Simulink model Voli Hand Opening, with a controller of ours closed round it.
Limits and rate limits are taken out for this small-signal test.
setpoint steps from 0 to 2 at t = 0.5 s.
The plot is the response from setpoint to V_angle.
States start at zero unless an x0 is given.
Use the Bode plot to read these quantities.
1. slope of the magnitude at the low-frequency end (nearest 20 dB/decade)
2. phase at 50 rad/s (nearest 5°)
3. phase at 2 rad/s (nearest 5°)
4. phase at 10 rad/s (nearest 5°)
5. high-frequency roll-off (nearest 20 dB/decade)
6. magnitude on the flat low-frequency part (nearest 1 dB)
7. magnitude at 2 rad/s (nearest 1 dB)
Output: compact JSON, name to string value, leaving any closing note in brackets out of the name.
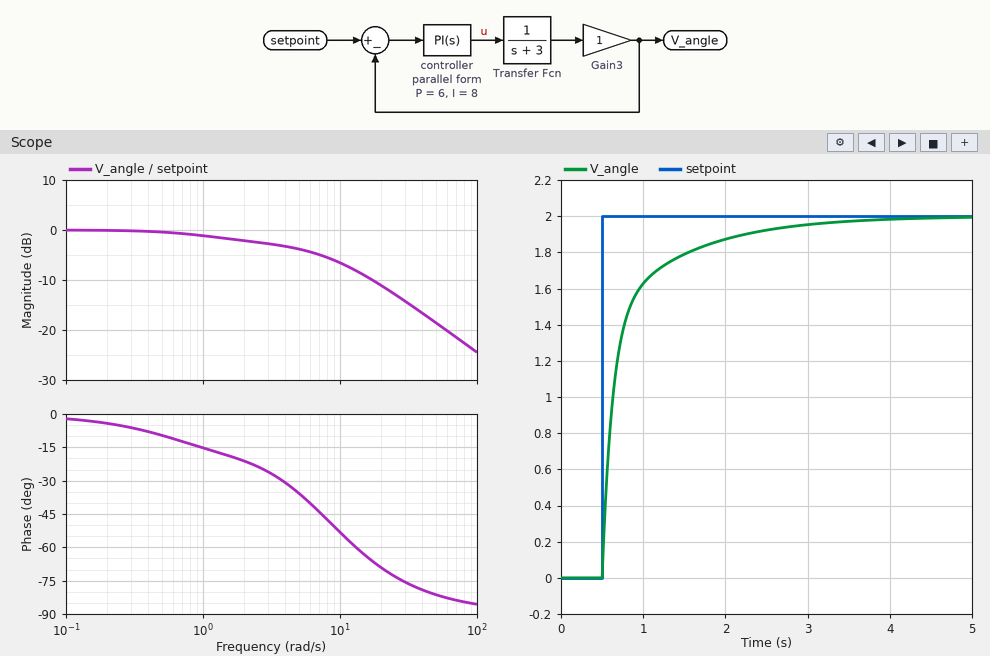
{"slope of the magnitude at the low-frequency end": "0 dB/decade", "phase at 50 rad/s": "-80°", "phase at 2 rad/s": "-20°", "phase at 10 rad/s": "-55°", "high-frequency roll-off": "-20 dB/decade", "magnitude on the flat low-frequency part": "0 dB", "magnitude at 2 rad/s": "-2 dB"}
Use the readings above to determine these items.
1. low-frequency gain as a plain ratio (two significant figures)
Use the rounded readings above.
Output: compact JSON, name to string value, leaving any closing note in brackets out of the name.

{"low-frequency gain as a plain ratio": "1.0"}
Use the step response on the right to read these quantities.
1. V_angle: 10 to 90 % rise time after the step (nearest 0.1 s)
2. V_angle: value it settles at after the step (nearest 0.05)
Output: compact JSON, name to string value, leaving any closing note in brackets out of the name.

{"V_angle: 10 to 90 % rise time after the step": "1.0 s", "V_angle: value it settles at after the step": "2.00"}
